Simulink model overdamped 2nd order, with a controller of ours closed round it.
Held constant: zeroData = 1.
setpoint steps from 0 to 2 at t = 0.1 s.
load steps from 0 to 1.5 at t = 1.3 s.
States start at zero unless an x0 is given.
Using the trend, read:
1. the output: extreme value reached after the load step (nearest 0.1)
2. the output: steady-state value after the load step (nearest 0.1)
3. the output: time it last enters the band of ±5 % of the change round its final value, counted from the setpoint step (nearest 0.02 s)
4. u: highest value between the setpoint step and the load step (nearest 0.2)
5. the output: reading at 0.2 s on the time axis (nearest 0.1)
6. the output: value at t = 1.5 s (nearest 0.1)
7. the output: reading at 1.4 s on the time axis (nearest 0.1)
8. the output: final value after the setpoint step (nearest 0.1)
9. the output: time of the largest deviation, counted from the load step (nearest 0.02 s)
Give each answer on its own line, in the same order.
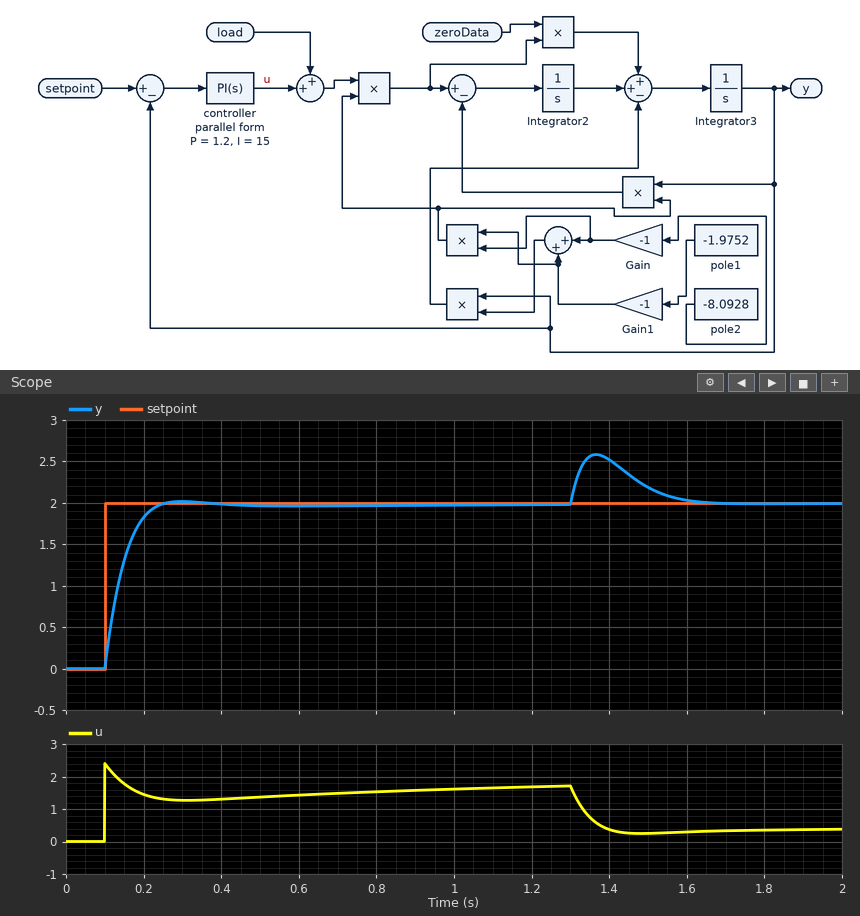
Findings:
2.6
2.0
0.12 s
2.4
1.8
2.2
2.5
2.0
0.06 s
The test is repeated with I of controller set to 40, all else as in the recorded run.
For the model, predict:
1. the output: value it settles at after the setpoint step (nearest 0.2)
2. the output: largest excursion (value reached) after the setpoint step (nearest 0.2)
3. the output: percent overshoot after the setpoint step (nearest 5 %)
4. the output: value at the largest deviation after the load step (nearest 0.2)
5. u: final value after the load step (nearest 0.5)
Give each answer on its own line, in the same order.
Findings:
2.0
2.4
15 %
2.4
0.5
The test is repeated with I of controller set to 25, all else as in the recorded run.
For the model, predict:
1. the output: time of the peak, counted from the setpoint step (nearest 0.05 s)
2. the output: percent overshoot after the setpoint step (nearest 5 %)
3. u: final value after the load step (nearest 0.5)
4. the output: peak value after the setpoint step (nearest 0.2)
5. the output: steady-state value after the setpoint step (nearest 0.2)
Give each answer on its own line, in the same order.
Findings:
0.15 s
10 %
0.5
2.2
2.0
